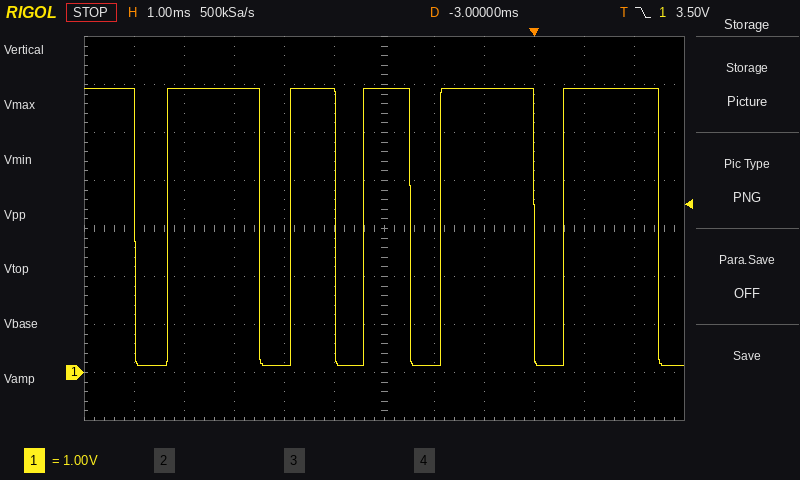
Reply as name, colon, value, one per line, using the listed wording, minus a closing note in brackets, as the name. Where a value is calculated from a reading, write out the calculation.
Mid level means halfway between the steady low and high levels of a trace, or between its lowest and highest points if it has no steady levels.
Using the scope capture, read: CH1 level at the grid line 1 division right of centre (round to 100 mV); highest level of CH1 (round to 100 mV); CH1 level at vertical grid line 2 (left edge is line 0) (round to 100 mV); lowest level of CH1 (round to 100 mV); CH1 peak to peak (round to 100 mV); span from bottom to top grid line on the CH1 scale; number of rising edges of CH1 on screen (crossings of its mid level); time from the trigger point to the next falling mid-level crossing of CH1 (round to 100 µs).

CH1 level at the grid line 1 division right of centre: 100 mV
highest level of CH1: 5.9 V
CH1 level at vertical grid line 2 (left edge is line 0): 5.9 V
lowest level of CH1: 100 mV
CH1 peak to peak: 5.9 V − (100 mV) = 5.8 V
span from bottom to top grid line on the CH1 scale: 8 V
number of rising edges of CH1 on screen: 5
time from the trigger point to the next falling mid-level crossing of CH1: 2.5 ms
